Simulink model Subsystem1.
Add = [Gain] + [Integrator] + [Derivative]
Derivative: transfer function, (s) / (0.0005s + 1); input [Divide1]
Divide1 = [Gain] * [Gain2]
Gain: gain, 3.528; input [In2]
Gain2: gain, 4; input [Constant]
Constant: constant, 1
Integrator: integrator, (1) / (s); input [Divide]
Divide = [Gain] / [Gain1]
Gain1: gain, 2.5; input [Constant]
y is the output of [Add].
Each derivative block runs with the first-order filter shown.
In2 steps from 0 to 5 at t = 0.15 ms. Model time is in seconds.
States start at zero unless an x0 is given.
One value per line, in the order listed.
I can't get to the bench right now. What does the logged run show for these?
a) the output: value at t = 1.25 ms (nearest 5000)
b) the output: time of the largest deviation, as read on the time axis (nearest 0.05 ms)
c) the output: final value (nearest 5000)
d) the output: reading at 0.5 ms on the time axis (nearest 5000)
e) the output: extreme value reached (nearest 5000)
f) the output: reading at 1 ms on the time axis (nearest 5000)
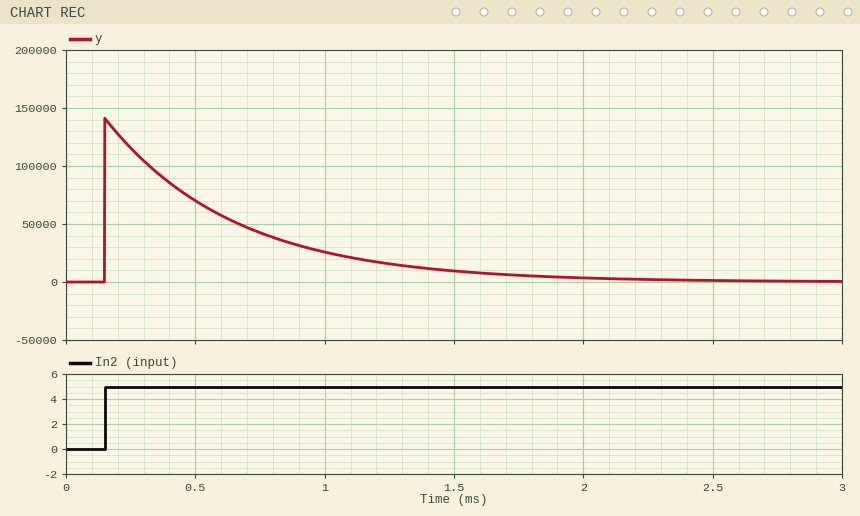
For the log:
15000
0.15 ms
0
70000
140000
25000
